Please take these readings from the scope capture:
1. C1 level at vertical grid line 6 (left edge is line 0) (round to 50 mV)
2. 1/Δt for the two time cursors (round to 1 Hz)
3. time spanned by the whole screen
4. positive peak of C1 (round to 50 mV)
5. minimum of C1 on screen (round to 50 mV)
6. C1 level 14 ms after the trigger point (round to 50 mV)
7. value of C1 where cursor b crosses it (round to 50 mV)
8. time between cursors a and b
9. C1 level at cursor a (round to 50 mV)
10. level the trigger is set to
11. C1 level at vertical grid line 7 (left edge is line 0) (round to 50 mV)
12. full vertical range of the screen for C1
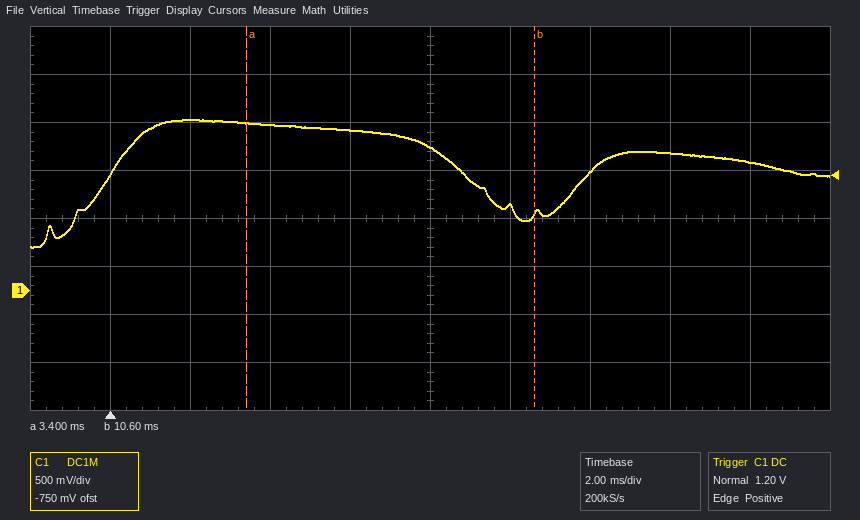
850 mV
139 Hz
20 ms
1.80 V
450 mV
1.45 V
800 mV
7.2 ms
1.75 V
1.20 V
1.25 V
4 V
